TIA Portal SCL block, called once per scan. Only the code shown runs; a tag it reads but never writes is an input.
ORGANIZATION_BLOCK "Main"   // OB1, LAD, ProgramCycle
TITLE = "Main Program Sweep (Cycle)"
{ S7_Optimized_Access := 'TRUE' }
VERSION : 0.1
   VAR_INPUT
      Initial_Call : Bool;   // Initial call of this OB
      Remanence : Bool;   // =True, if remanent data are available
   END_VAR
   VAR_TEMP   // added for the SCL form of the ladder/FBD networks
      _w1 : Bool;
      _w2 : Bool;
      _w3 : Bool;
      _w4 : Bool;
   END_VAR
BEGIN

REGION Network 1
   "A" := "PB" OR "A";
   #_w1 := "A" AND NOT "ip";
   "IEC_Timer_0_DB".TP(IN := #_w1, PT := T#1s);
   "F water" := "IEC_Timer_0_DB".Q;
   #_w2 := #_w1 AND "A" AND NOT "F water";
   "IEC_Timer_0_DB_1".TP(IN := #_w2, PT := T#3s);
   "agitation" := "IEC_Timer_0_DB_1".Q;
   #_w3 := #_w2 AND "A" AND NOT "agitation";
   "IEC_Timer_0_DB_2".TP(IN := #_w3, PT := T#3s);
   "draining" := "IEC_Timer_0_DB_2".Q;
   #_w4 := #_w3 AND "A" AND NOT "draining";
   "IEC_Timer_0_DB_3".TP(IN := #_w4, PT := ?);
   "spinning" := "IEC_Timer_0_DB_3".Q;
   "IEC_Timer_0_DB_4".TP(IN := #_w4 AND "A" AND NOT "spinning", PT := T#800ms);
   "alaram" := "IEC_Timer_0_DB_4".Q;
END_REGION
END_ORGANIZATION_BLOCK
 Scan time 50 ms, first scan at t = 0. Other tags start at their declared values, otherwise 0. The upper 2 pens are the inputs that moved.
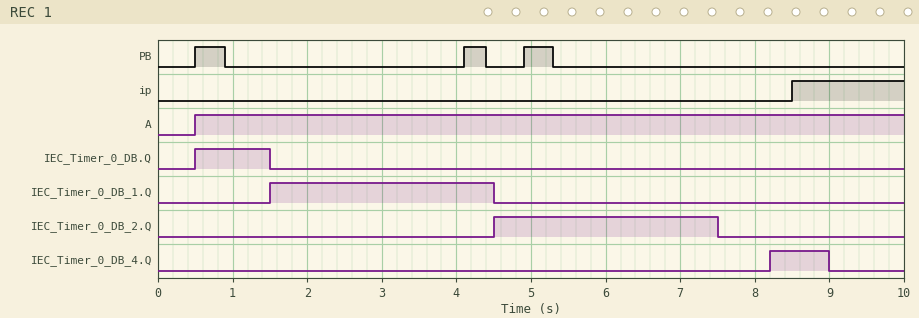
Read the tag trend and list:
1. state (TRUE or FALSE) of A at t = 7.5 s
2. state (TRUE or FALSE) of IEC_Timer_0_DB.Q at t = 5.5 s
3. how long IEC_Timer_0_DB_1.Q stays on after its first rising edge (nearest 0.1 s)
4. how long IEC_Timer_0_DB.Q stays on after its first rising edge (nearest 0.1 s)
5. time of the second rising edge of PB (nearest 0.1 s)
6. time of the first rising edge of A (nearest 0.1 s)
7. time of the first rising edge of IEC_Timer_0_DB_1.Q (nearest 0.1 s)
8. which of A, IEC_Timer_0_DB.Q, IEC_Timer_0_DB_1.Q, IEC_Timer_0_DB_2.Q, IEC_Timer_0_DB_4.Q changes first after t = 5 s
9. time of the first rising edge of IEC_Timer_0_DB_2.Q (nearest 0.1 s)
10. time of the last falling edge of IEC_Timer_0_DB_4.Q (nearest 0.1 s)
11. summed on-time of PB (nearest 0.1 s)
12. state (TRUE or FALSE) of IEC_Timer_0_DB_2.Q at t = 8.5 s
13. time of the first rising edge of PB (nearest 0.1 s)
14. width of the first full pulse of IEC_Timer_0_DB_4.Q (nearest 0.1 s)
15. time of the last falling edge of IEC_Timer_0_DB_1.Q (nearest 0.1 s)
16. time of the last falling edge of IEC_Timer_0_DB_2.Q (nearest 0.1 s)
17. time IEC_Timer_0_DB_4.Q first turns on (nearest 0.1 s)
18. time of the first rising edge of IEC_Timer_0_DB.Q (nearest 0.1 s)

TRUE
FALSE
3.0 s
1.0 s
4.1 s
0.5 s
1.5 s
IEC_Timer_0_DB_2.Q
4.5 s
9.0 s
1.1 s
FALSE
0.5 s
0.8 s
4.5 s
7.5 s
8.2 s
0.5 s
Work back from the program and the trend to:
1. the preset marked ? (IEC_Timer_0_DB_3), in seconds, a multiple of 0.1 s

0.7 s
